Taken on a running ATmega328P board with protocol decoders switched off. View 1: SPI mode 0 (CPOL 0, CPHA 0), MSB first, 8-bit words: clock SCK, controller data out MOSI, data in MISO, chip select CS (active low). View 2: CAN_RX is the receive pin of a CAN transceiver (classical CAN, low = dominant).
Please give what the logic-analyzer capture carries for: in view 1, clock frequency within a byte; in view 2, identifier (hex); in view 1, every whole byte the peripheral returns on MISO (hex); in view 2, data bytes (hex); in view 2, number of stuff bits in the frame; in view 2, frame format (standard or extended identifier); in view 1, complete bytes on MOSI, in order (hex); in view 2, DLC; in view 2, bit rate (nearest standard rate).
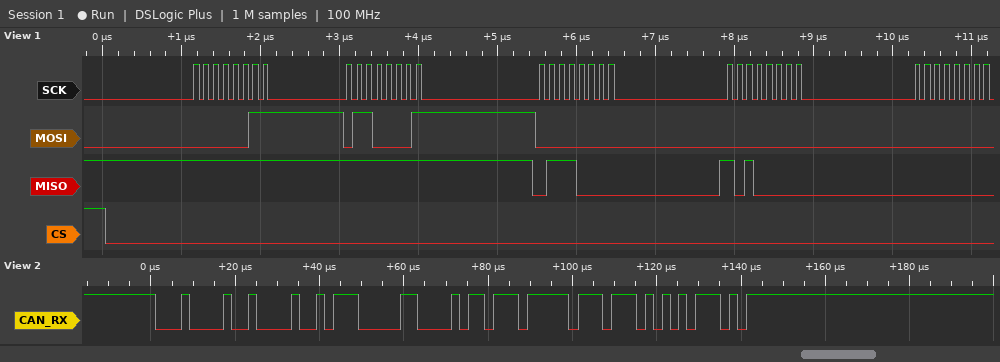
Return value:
8 MHz
0x109
0xFF 0xFF 0x70 0xA0 0x00
B8 21 6E FF
2
standard
0x03 0x61 0x00 0x00 0x00
4
500 kbit/s
